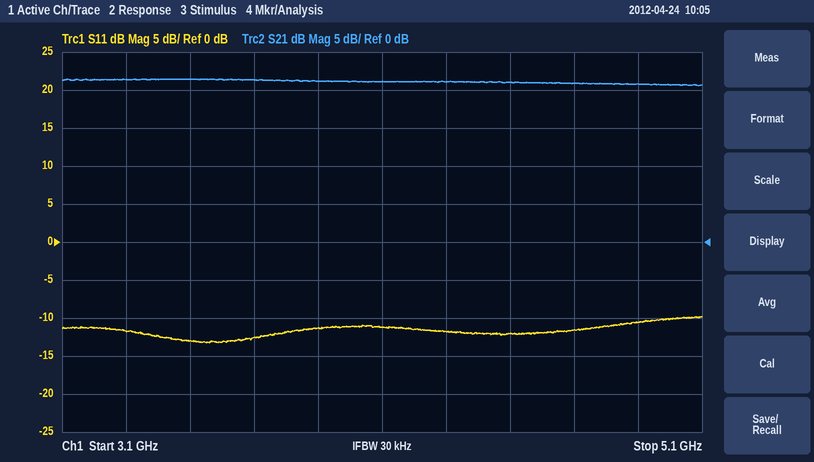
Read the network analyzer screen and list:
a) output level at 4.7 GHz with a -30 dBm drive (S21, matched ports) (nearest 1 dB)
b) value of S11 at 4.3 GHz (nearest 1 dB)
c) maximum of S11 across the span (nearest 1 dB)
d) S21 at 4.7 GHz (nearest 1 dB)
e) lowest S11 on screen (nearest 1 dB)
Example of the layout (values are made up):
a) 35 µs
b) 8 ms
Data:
a) -9 dBm
b) -12 dB
c) -10 dB
d) 21 dB
e) -13 dB
